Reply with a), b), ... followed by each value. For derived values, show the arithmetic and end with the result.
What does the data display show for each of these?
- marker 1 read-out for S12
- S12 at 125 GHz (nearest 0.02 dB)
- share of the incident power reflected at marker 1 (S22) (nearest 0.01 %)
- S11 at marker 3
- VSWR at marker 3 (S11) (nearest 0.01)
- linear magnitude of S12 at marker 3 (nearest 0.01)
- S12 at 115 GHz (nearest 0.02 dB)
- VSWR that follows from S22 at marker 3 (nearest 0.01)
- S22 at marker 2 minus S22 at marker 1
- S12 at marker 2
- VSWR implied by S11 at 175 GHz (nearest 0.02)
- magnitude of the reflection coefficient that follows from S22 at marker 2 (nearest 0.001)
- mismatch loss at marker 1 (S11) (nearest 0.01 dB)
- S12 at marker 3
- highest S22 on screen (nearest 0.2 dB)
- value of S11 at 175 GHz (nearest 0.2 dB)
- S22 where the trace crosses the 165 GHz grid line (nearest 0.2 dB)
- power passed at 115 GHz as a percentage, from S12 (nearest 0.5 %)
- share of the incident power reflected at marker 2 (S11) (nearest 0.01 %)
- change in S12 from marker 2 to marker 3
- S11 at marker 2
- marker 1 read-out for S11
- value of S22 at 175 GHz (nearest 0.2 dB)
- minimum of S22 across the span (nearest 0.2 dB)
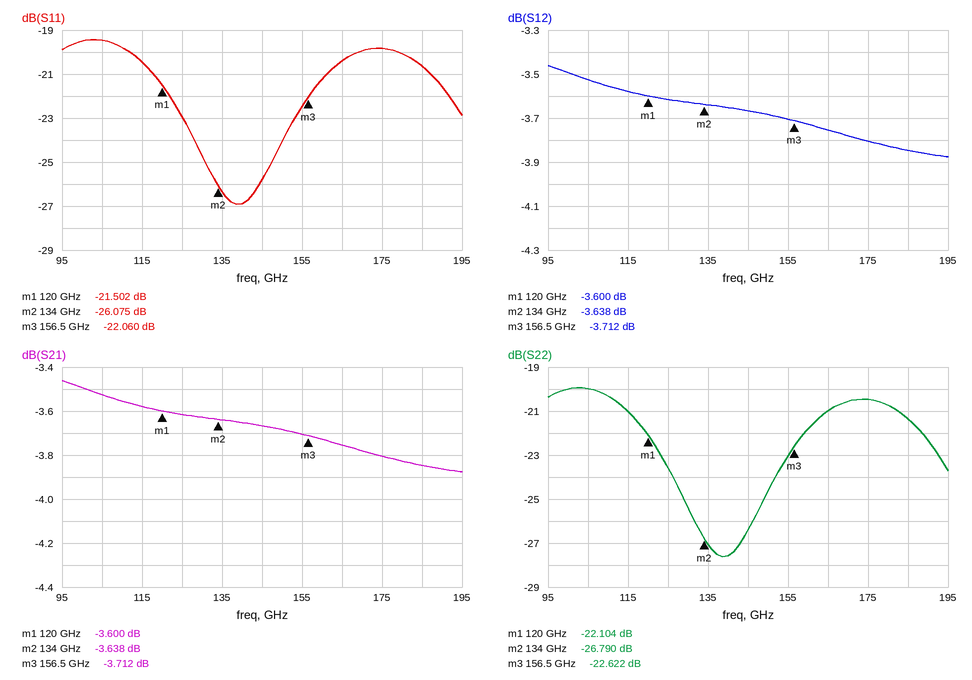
a) -3.600 dB
b) -3.62 dB
c) 10^(-22.104/10) ≈ 0.62 %
d) -22.060 dB
e) (1 + 0.0789)/(1 − 0.0789) ≈ 1.17
f) 10^(-3.712/20) ≈ 0.65
g) -3.58 dB
h) (1 + 0.0739)/(1 − 0.0739) ≈ 1.16
i) -26.79 − (-22.104) = -4.686 dB
j) -3.638 dB
k) |Γ| = 10^(-19.8/20) = 0.1023; VSWR = (1 + 0.1023)/(1 − 0.1023) ≈ 1.23, so 1.22 to the nearest 0.02
l) 10^(-26.79/20) ≈ 0.046
m) −10 log10(1 − 10^(-21.502/10)) ≈ 0.03 dB
n) -3.712 dB
o) -20.0 dB
p) -19.8 dB
q) -21.0 dB
r) 10^(-3.58/10) ≈ 43.9 %, so 44.0 % to the nearest 0.5 %
s) 10^(-26.075/10) ≈ 0.25 %
t) -3.712 − (-3.638) = -0.074 dB
u) -26.075 dB
v) -21.502 dB
w) -20.4 dB
x) -27.6 dB
